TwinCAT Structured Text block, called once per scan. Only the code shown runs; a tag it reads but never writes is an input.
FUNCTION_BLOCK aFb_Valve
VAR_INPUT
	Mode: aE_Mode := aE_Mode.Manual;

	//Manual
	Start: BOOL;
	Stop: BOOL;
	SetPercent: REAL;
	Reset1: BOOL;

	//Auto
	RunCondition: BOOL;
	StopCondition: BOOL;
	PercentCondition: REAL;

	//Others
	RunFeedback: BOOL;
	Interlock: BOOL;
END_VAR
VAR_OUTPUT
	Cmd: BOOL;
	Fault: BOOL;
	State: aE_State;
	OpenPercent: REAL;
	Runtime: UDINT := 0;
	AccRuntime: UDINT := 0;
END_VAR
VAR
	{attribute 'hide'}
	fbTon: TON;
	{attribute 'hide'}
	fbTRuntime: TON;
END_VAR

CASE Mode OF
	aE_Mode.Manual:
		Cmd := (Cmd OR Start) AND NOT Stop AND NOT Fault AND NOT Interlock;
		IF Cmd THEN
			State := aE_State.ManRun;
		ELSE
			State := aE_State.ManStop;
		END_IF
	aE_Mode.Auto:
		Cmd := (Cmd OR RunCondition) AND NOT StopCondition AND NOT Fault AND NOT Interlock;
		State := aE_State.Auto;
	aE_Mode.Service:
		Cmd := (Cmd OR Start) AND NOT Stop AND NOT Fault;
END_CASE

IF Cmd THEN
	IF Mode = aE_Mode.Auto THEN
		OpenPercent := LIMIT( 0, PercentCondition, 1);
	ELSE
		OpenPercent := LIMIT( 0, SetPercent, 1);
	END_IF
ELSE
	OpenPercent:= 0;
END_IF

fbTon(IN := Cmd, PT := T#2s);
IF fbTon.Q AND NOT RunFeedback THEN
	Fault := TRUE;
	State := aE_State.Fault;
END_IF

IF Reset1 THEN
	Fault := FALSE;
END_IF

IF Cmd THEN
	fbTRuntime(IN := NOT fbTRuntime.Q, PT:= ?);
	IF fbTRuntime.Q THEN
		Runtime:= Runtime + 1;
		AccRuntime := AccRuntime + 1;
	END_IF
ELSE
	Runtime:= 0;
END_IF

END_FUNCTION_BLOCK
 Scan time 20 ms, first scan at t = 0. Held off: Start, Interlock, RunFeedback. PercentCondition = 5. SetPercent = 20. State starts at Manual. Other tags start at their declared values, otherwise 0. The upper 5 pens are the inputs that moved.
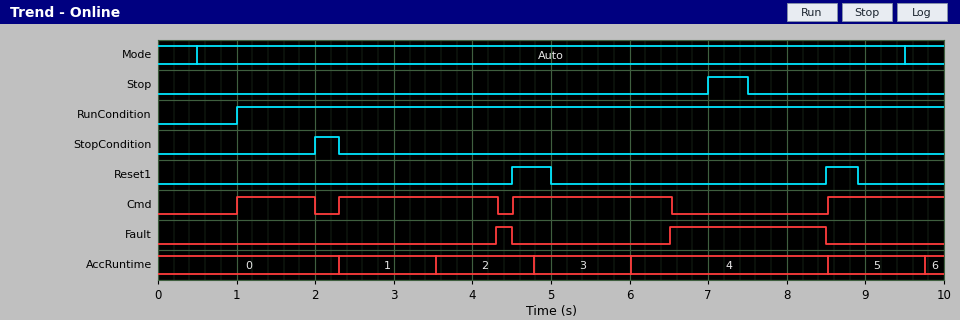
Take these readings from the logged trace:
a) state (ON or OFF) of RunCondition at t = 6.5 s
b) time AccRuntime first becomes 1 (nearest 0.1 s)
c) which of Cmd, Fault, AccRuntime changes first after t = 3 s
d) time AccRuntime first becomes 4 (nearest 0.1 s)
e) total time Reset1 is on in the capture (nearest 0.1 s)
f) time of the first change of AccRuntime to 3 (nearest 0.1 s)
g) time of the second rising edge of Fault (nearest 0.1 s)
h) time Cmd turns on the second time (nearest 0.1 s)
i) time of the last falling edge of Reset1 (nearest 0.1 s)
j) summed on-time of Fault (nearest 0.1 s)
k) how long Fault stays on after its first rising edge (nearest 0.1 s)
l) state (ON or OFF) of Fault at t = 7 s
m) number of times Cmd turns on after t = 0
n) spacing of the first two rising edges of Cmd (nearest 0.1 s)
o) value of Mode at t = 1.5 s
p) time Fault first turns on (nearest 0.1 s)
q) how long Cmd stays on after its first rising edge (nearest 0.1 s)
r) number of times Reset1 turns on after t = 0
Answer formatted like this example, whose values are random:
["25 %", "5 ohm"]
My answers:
["ON", "2.3 s", "AccRuntime", "6.0 s", "0.9 s", "4.8 s", "6.5 s", "2.3 s", "8.9 s", "2.2 s", "0.2 s", "ON", "4", "1.3 s", "Auto", "4.3 s", "1.0 s", "2"]
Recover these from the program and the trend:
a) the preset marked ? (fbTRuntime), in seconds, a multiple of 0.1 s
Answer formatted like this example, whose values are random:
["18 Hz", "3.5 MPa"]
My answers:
["1.2 s"]
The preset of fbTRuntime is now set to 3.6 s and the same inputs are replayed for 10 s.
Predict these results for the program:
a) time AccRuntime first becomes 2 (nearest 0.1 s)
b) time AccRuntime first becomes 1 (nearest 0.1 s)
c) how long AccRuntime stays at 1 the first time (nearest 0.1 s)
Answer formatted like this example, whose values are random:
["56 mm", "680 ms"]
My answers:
["8.5 s", "4.6 s", "3.9 s"]
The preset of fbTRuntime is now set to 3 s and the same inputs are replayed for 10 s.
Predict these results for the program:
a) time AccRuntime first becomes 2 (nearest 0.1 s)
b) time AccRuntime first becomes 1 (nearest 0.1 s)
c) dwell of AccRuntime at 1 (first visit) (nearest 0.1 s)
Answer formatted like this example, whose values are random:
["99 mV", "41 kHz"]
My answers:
["8.5 s", "4.0 s", "4.5 s"]
